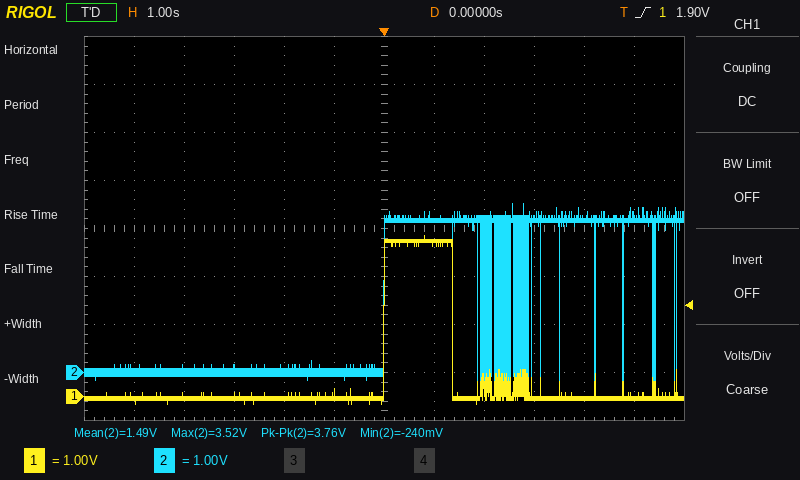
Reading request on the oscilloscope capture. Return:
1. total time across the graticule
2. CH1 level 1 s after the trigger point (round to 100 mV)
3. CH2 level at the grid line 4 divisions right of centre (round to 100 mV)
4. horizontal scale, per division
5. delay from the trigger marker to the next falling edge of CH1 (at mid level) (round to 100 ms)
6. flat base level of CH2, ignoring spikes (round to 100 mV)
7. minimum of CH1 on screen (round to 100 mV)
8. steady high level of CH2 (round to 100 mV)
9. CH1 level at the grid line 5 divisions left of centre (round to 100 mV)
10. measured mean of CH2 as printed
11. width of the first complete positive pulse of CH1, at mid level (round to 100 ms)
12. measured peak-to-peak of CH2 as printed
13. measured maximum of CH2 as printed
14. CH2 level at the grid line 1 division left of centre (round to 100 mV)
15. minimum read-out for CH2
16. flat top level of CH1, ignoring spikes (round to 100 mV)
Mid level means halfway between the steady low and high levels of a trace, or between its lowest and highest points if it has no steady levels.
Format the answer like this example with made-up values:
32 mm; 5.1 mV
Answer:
12 s; 3.2 V; 3.2 V; 1 s; 1.4 s; 0.0 V; -200 mV; 3.2 V; -100 mV; 1.49 V; 1.4 s; 3.76 V; 3.52 V; 0.0 V; -240 mV; 3.2 V
